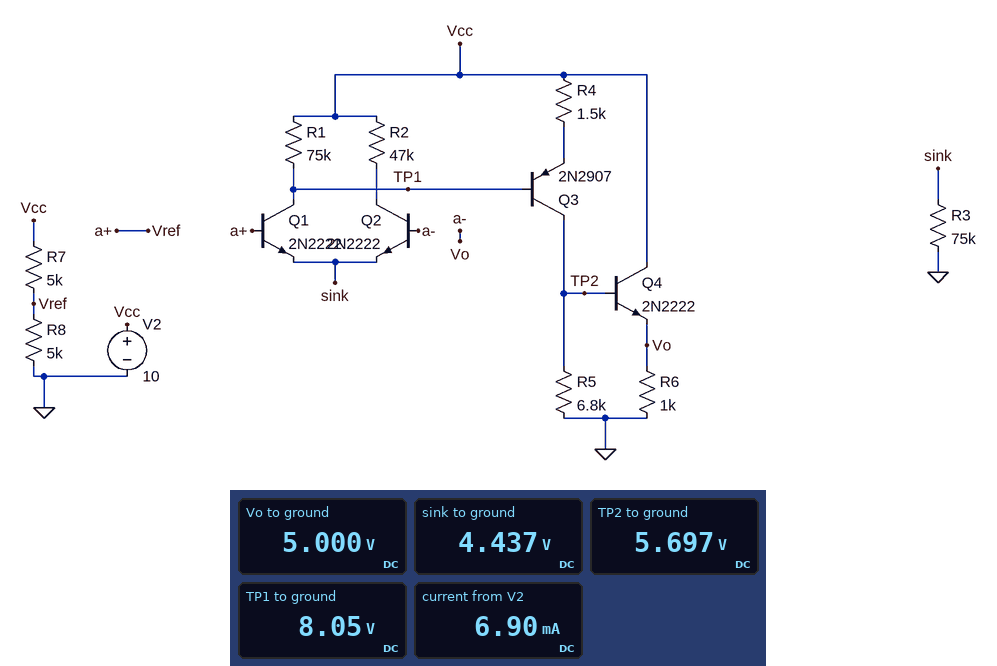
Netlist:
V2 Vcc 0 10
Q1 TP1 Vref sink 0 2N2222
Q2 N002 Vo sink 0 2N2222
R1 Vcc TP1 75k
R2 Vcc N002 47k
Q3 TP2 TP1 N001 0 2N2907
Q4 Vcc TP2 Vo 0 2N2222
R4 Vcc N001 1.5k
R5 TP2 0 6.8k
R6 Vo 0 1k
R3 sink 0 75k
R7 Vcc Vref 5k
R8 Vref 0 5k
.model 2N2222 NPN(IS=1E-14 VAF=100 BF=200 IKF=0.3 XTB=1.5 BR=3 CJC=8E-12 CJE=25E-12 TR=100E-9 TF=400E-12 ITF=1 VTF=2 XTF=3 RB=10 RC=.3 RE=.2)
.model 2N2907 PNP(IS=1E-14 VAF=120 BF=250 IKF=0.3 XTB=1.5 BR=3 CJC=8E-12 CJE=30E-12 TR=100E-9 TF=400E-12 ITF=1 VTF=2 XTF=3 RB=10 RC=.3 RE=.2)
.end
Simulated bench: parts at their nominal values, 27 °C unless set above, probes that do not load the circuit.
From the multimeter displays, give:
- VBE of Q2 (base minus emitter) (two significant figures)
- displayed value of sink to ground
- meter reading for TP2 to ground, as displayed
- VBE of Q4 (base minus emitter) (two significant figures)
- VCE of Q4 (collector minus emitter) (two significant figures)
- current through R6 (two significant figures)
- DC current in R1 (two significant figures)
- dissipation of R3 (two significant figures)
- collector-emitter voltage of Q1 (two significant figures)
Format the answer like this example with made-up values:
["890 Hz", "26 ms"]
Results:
["560 mV", "4.437 V", "5.697 V", "700 mV", "5.0 V", "5.0 mA", "26 µA", "260 µW", "3.6 V"]
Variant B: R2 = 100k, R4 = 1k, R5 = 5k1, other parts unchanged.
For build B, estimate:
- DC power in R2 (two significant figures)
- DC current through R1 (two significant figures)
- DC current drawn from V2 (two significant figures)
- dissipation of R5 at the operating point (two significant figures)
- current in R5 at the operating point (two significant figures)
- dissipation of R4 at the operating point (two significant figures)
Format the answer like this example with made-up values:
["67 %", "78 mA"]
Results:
["92 µW", "24 µA", "7.2 mA", "6.4 mW", "1.1 mA", "1.3 mW"]
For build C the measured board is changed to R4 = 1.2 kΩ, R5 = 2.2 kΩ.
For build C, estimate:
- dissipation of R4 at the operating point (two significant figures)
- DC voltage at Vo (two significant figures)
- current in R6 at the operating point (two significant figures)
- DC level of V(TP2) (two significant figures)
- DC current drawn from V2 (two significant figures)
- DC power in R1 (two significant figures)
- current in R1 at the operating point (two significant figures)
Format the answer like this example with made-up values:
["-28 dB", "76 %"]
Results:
["7.4 mW", "4.7 V", "4.7 mA", "5.4 V", "8.2 mA", "180 µW", "49 µA"]
